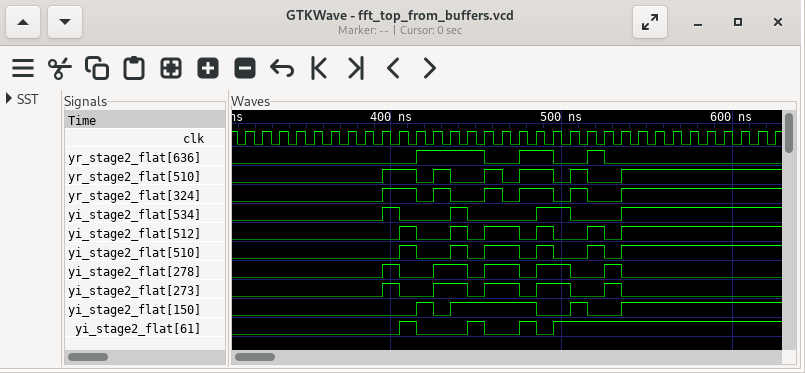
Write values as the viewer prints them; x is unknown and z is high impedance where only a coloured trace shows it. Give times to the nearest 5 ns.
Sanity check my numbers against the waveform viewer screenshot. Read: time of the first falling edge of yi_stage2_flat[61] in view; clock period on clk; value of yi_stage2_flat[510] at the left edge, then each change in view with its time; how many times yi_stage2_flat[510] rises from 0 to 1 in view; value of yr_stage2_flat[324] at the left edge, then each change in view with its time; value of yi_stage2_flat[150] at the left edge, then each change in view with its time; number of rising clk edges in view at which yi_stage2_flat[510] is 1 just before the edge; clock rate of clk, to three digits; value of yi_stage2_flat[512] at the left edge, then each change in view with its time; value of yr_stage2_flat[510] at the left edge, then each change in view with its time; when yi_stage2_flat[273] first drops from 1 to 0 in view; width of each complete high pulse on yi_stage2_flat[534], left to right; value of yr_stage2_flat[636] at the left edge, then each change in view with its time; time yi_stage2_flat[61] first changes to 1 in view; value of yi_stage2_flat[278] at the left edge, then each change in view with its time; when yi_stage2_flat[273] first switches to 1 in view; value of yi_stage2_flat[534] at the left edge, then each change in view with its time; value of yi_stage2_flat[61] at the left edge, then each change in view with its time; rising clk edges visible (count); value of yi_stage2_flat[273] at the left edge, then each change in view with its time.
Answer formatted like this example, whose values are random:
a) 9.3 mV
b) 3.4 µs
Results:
a) 415 ns
b) 10 ns
c) 0, 1 at 405 ns, 0 at 415 ns, 1 at 435 ns, 0 at 445 ns, 1 at 455 ns, 0 at 475 ns, 1 at 485 ns, 0 at 495 ns, 1 at 515 ns, 0 at 525 ns, 1 at 535 ns
d) 6
e) 0, 1 at 395 ns, 0 at 415 ns, 1 at 425 ns, 0 at 435 ns, 1 at 455 ns, 0 at 465 ns, 1 at 475 ns, 0 at 495 ns, 1 at 505 ns, 0 at 515 ns, 1 at 535 ns
f) 0, 1 at 415 ns, 0 at 425 ns, 1 at 435 ns, 0 at 485 ns, 1 at 505 ns, 0 at 515 ns, 1 at 535 ns
g) 15
h) 100 MHz
i) 0, 1 at 405 ns, 0 at 415 ns, 1 at 435 ns, 0 at 445 ns, 1 at 455 ns, 0 at 475 ns, 1 at 485 ns, 0 at 495 ns, 1 at 515 ns, 0 at 525 ns, 1 at 535 ns
j) 0, 1 at 395 ns, 0 at 415 ns, 1 at 425 ns, 0 at 435 ns, 1 at 455 ns, 0 at 465 ns, 1 at 475 ns, 0 at 495 ns, 1 at 505 ns, 0 at 515 ns, 1 at 535 ns
k) 405 ns
l) 10 ns, 10 ns, 20 ns
m) 0, 1 at 415 ns, 0 at 455 ns, 1 at 475 ns, 0 at 495 ns, 1 at 515 ns, 0 at 525 ns
n) 405 ns
o) 0, 1 at 395 ns, 0 at 405 ns, 1 at 425 ns, 0 at 445 ns, 1 at 455 ns, 0 at 475 ns, 1 at 485 ns, 0 at 505 ns, 1 at 525 ns, 0 at 535 ns
p) 395 ns
q) 0, 1 at 395 ns, 0 at 405 ns, 1 at 435 ns, 0 at 445 ns, 1 at 485 ns, 0 at 505 ns, 1 at 535 ns
r) 0, 1 at 405 ns, 0 at 415 ns, 1 at 445 ns, 0 at 455 ns, 1 at 475 ns, 0 at 485 ns, 1 at 495 ns
s) 32
t) 0, 1 at 395 ns, 0 at 405 ns, 1 at 425 ns, 0 at 445 ns, 1 at 455 ns, 0 at 475 ns, 1 at 485 ns, 0 at 505 ns, 1 at 525 ns, 0 at 535 ns
